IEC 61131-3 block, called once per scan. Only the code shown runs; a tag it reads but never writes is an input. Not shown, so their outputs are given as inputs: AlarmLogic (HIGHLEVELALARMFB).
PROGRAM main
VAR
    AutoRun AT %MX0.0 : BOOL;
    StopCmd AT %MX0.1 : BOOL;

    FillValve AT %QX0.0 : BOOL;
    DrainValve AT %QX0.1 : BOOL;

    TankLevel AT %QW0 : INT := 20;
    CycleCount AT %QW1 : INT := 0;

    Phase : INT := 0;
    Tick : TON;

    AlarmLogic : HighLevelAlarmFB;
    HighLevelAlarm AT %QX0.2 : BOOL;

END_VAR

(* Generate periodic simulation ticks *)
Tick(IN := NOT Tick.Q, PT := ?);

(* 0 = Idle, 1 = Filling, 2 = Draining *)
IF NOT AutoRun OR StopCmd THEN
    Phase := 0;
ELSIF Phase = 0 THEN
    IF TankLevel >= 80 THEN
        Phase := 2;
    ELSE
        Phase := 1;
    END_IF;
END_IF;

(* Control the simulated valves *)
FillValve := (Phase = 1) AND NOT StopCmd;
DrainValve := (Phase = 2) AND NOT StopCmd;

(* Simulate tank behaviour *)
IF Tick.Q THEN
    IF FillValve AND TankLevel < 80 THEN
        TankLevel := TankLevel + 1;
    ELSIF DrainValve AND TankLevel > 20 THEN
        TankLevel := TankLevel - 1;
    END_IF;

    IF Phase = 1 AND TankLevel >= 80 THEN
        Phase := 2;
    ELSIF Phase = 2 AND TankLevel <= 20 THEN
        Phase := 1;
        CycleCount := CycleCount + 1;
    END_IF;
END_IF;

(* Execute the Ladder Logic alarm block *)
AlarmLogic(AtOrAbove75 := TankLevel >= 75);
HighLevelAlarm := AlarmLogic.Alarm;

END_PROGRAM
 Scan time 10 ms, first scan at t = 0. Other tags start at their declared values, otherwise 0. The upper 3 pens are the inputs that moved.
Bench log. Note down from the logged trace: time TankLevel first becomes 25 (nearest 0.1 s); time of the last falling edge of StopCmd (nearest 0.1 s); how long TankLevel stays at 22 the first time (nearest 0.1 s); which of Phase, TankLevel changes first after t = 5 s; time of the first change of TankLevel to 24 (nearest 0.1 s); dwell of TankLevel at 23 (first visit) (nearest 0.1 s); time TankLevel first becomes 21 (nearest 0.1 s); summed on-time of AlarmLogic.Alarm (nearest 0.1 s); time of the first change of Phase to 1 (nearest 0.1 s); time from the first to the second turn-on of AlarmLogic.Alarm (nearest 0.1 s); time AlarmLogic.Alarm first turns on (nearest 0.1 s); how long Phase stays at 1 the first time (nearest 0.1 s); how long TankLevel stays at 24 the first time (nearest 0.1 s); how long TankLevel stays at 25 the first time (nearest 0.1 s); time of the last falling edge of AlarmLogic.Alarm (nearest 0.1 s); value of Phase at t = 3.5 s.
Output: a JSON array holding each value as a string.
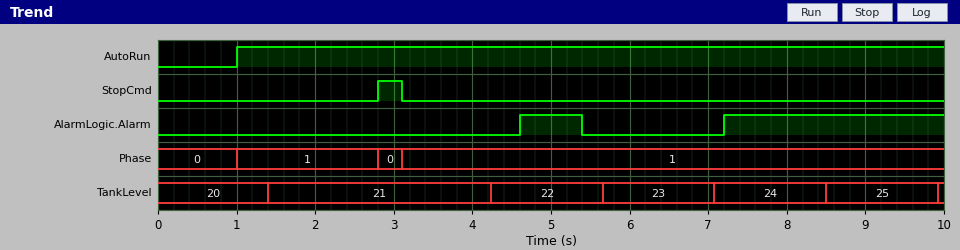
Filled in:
["8.5 s", "3.1 s", "1.4 s", "TankLevel", "7.1 s", "1.4 s", "1.4 s", "3.6 s", "1.0 s", "2.6 s", "4.6 s", "1.8 s", "1.4 s", "1.4 s", "5.4 s", "1"]
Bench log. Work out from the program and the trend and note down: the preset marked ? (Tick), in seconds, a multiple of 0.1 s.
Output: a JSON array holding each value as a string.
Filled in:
["1.4 s"]
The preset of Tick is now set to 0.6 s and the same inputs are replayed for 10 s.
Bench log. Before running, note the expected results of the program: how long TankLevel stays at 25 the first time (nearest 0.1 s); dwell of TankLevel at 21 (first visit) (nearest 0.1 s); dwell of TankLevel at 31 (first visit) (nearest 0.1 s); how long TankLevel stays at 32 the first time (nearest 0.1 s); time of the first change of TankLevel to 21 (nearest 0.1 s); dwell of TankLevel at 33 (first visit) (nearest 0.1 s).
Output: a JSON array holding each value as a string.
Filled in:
["0.6 s", "0.6 s", "0.6 s", "0.6 s", "1.2 s", "0.6 s"]
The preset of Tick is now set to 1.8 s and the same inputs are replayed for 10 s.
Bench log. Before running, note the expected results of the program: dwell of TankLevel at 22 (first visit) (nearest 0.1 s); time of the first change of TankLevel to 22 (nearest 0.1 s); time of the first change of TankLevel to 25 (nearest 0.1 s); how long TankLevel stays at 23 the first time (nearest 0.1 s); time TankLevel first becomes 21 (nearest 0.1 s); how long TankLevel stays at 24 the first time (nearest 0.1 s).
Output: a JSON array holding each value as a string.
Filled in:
["1.8 s", "3.6 s", "9.1 s", "1.8 s", "1.8 s", "1.8 s"]
